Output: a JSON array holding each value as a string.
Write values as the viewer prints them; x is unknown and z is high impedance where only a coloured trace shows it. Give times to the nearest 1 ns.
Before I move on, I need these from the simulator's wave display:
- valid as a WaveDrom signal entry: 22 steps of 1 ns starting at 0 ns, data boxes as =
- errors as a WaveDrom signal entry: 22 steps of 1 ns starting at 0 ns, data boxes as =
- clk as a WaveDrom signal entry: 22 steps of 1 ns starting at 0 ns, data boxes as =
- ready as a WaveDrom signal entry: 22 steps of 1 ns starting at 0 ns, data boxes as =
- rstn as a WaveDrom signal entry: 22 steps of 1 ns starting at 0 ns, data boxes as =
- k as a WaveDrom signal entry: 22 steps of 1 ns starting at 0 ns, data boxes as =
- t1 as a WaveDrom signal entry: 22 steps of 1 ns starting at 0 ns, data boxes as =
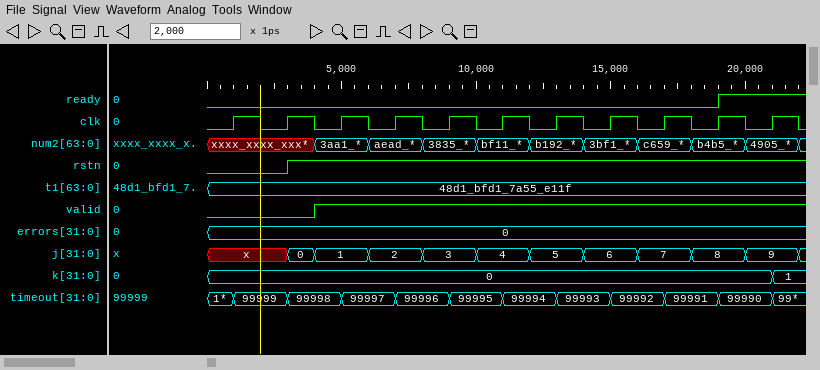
["{name: 'valid', wave: '0...1.................'}", "{name: 'errors', wave: '=.....................', data: '0'}", "{name: 'clk', wave: '0101010101010101010101'}", "{name: 'ready', wave: '0..................1..'}", "{name: 'rstn', wave: '0..1..................'}", "{name: 'k', wave: '=....................=', data: '0 1'}", "{name: 't1', wave: '=.....................', data: '48d1_bfd1_7a55_e11f'}"]
